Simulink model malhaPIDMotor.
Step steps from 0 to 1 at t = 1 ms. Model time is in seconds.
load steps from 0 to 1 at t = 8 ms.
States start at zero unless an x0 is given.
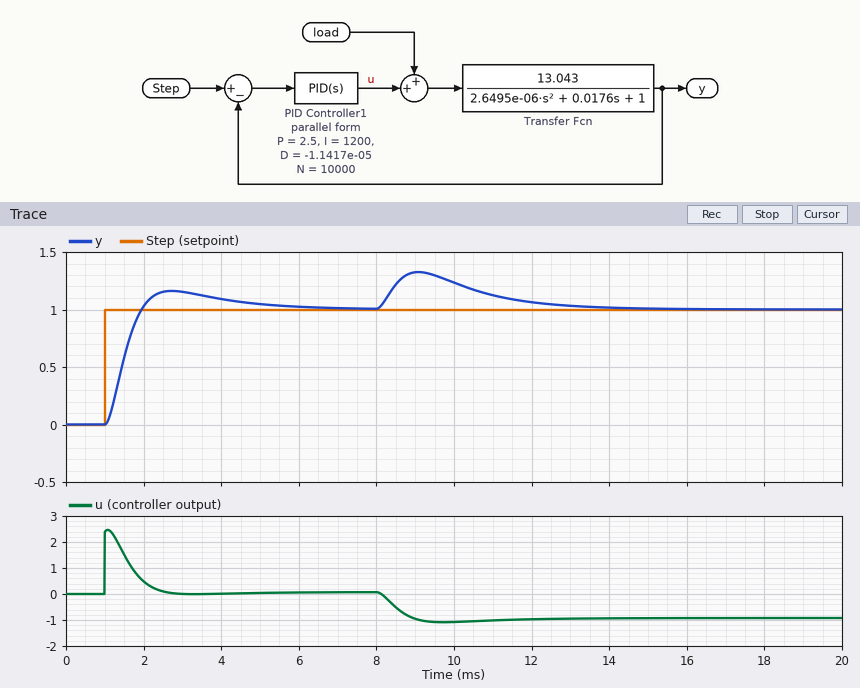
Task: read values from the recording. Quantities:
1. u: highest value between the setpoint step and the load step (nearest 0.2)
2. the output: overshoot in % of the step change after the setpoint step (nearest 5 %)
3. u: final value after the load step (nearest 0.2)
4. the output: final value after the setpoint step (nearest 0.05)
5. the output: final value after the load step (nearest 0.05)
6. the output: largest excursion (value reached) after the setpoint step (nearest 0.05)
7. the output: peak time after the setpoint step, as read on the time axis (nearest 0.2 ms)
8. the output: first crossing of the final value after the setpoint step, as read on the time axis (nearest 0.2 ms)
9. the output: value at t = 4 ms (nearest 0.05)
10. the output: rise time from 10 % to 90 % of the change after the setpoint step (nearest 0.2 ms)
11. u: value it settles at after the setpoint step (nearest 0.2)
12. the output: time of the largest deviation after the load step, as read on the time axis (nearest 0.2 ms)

2.4
15 %
-1.0
1.00
1.00
1.15
2.8 ms
2.0 ms
1.10
0.6 ms
0.0
9.0 ms
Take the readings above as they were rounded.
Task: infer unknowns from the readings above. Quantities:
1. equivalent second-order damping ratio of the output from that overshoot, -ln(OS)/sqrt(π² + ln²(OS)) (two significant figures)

0.52
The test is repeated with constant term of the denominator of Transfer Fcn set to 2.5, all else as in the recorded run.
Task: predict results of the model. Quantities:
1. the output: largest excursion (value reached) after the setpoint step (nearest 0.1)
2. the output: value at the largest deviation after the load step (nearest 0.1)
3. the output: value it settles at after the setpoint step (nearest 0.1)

1.1
1.3
1.0
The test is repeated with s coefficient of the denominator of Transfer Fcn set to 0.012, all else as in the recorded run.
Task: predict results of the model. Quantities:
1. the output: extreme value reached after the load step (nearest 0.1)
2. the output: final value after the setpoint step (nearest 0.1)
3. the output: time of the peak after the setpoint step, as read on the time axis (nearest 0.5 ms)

1.4
1.0
2.0 ms
